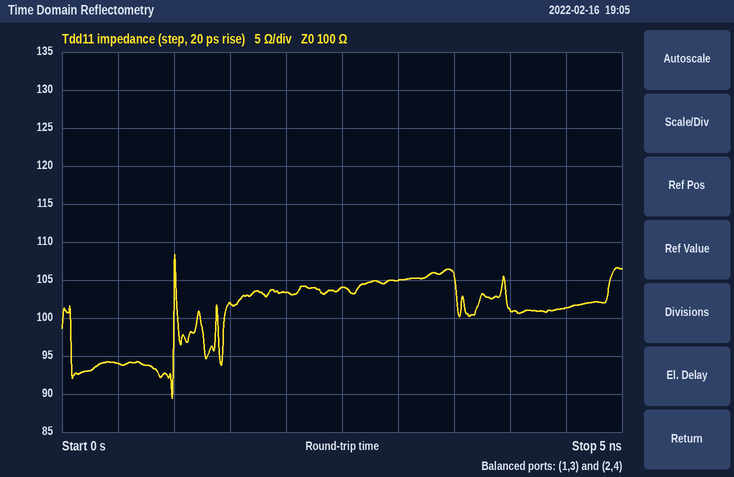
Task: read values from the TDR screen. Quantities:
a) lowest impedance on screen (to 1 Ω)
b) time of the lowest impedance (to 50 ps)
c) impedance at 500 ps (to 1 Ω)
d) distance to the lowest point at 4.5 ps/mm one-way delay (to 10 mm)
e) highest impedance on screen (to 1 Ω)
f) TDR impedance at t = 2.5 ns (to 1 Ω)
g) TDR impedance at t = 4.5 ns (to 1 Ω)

89 Ω
1.00 ns
94 Ω
110 mm
108 Ω
104 Ω
101 Ω
